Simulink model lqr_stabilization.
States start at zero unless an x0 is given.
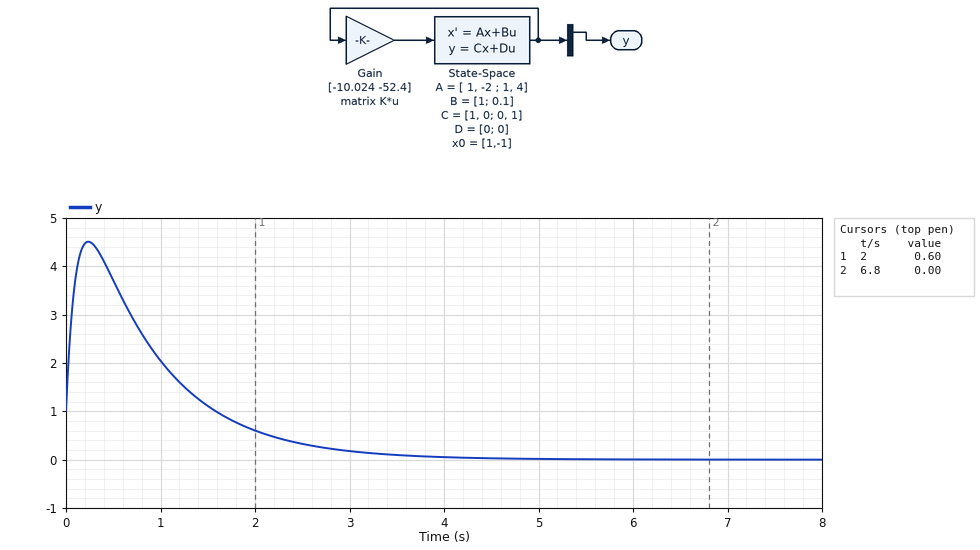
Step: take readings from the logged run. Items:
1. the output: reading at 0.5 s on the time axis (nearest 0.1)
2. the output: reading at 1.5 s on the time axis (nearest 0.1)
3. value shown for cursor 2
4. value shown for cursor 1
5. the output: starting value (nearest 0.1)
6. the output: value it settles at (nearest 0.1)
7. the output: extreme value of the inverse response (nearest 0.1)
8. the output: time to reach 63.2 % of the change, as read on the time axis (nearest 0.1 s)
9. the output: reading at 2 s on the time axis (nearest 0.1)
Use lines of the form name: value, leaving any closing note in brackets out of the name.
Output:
the output: reading at 0.5 s on the time axis: 3.7
the output: reading at 1.5 s on the time axis: 1.1
value shown for cursor 2: 0.00
value shown for cursor 1: 0.60
the output: starting value: 1.0
the output: value it settles at: 0.0
the output: extreme value of the inverse response: 4.5
the output: time to reach 63.2 % of the change, as read on the time axis: 2.4 s
the output: reading at 2 s on the time axis: 0.6
